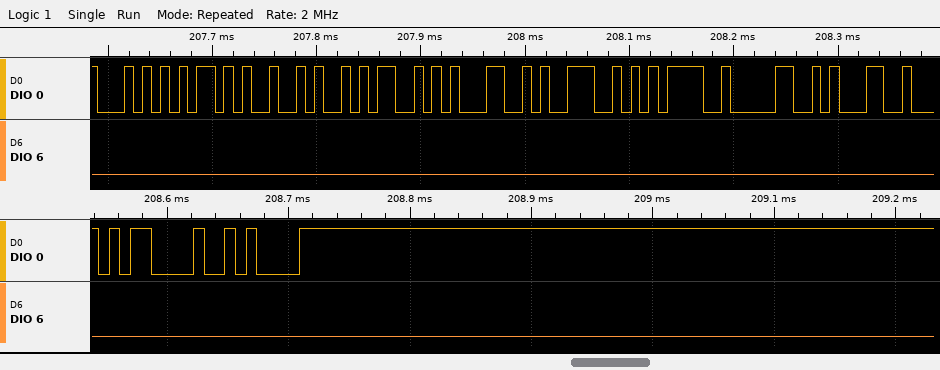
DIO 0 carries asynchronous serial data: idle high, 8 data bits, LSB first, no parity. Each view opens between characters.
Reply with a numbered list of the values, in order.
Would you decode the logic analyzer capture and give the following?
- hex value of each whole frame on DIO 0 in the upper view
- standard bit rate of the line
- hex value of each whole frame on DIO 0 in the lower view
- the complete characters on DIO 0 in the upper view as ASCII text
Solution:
1. 54, 2B, 4A, 53, 4C, 4E, 3D, 30, 31
2. 115200 baud
3. 0D, 0A
4. "T+JSLN=01"
